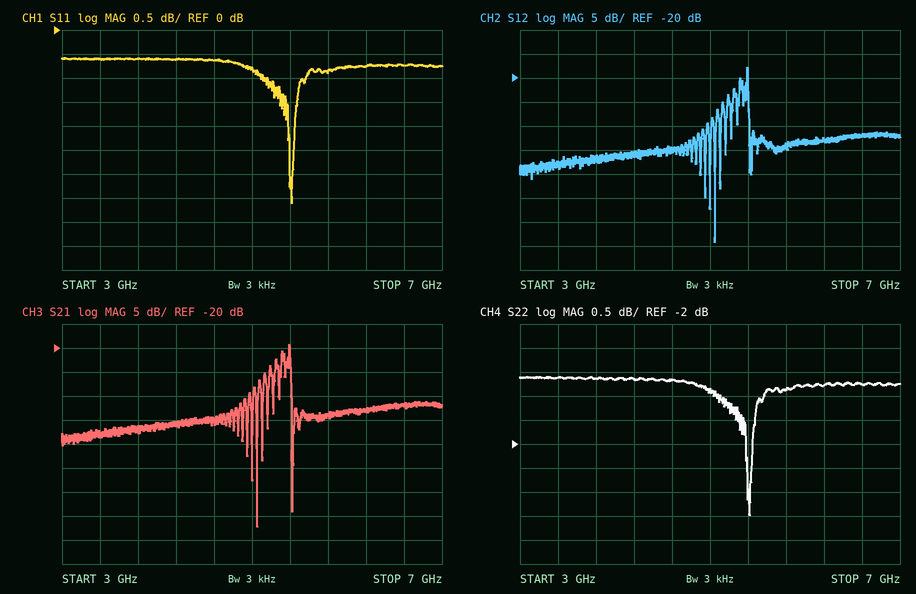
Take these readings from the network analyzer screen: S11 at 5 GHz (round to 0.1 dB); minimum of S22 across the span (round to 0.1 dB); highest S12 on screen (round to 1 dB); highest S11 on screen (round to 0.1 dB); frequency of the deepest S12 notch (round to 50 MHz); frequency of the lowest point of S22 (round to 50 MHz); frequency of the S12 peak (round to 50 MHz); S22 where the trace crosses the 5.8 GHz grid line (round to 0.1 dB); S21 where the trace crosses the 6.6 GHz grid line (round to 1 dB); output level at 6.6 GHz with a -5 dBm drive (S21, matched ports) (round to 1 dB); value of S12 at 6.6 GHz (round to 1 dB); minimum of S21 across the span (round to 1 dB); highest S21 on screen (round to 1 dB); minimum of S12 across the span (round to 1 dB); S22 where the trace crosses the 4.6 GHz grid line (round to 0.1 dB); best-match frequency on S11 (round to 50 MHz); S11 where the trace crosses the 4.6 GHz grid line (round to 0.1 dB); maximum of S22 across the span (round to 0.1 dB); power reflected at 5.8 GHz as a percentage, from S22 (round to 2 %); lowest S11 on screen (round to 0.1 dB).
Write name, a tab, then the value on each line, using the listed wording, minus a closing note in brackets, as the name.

S11 at 5 GHz	-0.8 dB
minimum of S22 across the span	-3.5 dB
highest S12 on screen	-18 dB
highest S11 on screen	-0.6 dB
frequency of the deepest S12 notch	5.05 GHz
frequency of the lowest point of S22	5.40 GHz
frequency of the S12 peak	5.40 GHz
S22 where the trace crosses the 5.8 GHz grid line	-0.9 dB
S21 where the trace crosses the 6.6 GHz grid line	-32 dB
output level at 6.6 GHz with a -5 dBm drive (S21, matched ports)	-37 dBm
value of S12 at 6.6 GHz	-32 dB
minimum of S21 across the span	-57 dB
highest S21 on screen	-19 dB
minimum of S12 across the span	-54 dB
S22 where the trace crosses the 4.6 GHz grid line	-0.7 dB
best-match frequency on S11	5.40 GHz
S11 where the trace crosses the 4.6 GHz grid line	-0.6 dB
maximum of S22 across the span	-0.6 dB
power reflected at 5.8 GHz as a percentage, from S22	82 %
lowest S11 on screen	-3.6 dB
